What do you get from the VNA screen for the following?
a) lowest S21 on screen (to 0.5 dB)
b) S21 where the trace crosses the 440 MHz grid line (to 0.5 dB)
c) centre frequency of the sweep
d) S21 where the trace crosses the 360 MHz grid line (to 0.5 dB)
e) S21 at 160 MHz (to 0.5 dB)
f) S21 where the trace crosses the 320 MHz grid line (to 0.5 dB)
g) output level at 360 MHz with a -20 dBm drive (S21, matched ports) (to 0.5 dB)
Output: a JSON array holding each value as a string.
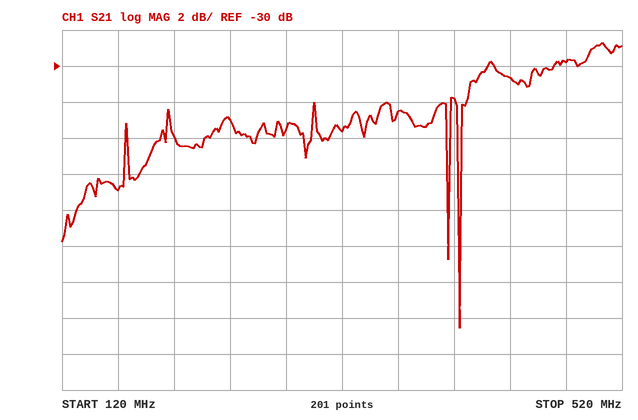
["-44.5 dB", "-30.5 dB", "320 MHz", "-32.5 dB", "-37.0 dB", "-33.5 dB", "-52.5 dBm"]
